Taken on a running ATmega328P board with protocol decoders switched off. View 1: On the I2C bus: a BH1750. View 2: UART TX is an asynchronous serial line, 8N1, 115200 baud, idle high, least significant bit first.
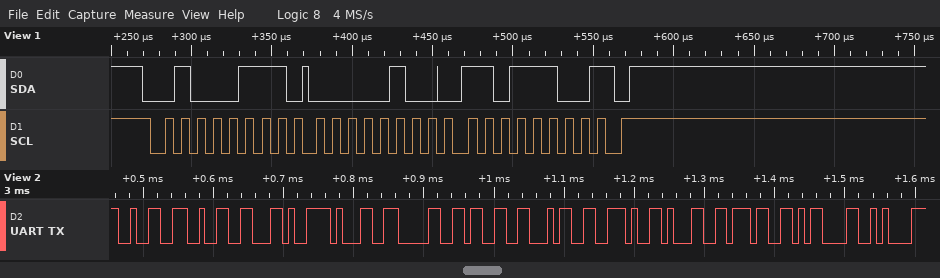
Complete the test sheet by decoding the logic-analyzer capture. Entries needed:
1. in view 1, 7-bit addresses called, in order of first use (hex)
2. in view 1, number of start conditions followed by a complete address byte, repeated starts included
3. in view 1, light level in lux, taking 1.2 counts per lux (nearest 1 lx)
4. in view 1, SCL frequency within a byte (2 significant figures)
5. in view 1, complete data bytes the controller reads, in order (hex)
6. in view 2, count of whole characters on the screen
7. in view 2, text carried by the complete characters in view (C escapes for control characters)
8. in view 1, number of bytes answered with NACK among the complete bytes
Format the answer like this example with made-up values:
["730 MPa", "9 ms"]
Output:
["0x23", "1", "1037 lx", "100 kHz", "04 DC", "12", "\"22,1034.17\\r\\n\"", "1"]
